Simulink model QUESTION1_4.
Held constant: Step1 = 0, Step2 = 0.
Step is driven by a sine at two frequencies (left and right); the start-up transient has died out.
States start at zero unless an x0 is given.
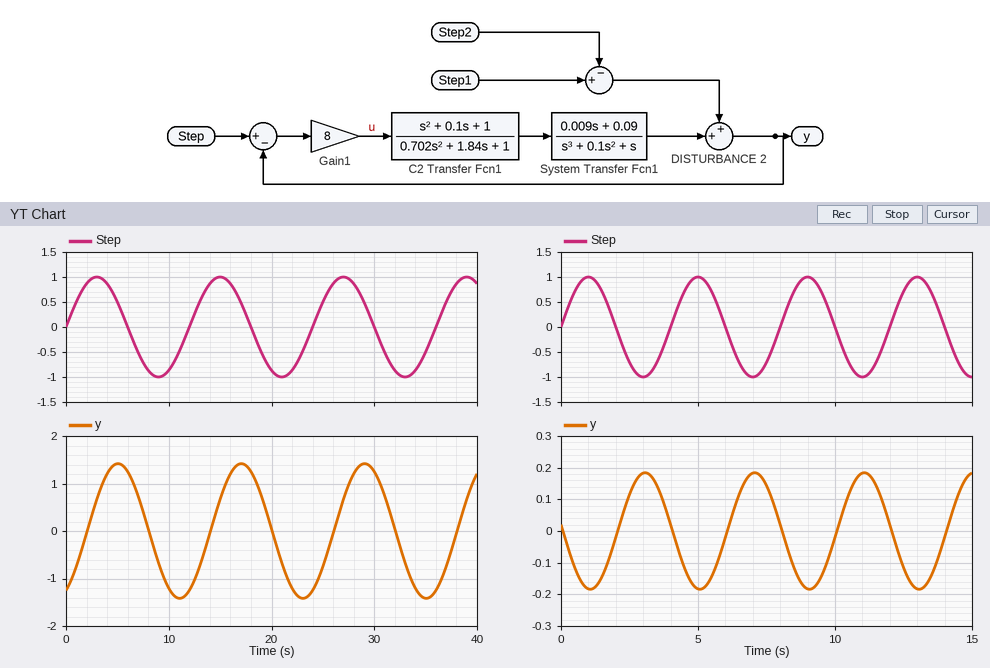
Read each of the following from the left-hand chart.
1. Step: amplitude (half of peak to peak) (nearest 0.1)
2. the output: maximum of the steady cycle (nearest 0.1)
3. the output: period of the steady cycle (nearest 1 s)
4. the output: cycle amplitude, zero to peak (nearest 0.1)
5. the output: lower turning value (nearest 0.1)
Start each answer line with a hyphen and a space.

- 1.0
- 1.4
- 12 s
- 1.4
- -1.4
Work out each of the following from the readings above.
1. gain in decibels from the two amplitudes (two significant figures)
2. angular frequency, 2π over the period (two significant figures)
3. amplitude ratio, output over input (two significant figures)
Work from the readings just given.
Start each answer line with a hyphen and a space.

- 2.9 dB
- 0.52 rad/s
- 1.4
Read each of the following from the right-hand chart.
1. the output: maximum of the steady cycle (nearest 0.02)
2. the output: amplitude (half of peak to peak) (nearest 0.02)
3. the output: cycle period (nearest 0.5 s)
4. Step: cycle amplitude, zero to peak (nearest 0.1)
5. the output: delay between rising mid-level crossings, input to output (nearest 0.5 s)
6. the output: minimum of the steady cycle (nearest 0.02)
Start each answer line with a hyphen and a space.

- 0.18
- 0.18
- 4.0 s
- 1.0
- 2.0 s
- -0.18
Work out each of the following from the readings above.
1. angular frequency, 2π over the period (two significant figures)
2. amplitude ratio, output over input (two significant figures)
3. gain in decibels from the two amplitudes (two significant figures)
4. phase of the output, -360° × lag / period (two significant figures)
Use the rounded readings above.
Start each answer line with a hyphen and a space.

- 1.6 rad/s
- 0.18
- -15 dB
- -180°
